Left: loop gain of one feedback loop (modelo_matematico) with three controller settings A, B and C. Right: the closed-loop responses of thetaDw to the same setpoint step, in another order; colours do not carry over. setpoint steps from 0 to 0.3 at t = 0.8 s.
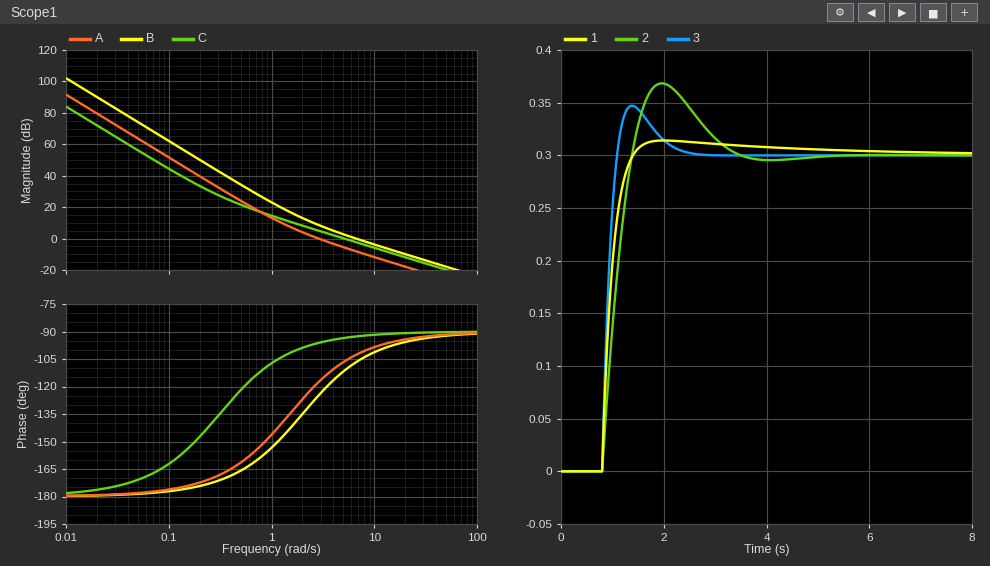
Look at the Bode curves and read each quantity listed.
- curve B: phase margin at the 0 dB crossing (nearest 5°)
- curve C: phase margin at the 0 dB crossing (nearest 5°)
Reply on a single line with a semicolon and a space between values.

75°; 85°
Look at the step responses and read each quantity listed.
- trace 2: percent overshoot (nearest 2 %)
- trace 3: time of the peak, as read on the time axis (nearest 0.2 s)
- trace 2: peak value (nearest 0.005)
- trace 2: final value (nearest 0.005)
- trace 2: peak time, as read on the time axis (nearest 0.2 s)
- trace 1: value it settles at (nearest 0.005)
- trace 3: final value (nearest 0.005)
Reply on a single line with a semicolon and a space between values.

22 %; 1.4 s; 0.370; 0.300; 2.0 s; 0.300; 0.300
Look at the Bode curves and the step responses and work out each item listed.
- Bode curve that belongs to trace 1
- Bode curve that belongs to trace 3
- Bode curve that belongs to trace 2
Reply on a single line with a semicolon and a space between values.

C; B; A
